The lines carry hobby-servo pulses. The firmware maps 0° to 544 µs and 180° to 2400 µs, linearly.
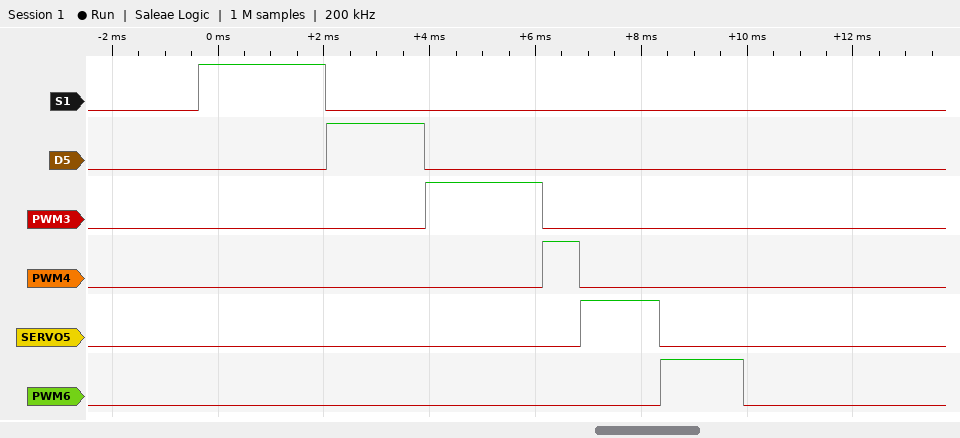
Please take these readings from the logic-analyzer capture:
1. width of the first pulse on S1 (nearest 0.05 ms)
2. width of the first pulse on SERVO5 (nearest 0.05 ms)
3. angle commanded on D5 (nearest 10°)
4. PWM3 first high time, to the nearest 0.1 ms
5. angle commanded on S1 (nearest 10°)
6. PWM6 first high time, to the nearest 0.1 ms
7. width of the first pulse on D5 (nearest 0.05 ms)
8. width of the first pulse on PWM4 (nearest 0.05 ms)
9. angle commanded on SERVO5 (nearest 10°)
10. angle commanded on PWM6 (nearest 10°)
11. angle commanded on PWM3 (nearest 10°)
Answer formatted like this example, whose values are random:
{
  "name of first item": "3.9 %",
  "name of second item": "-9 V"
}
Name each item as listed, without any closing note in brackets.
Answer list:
{
  "width of the first pulse on S1": "2.40 ms",
  "width of the first pulse on SERVO5": "1.50 ms",
  "angle commanded on D5": "130°",
  "PWM3 first high time, to the nearest 0.1 ms": "2.2 ms",
  "angle commanded on S1": "180°",
  "PWM6 first high time, to the nearest 0.1 ms": "1.6 ms",
  "width of the first pulse on D5": "1.85 ms",
  "width of the first pulse on PWM4": "0.70 ms",
  "angle commanded on SERVO5": "90°",
  "angle commanded on PWM6": "100°",
  "angle commanded on PWM3": "160°"
}
